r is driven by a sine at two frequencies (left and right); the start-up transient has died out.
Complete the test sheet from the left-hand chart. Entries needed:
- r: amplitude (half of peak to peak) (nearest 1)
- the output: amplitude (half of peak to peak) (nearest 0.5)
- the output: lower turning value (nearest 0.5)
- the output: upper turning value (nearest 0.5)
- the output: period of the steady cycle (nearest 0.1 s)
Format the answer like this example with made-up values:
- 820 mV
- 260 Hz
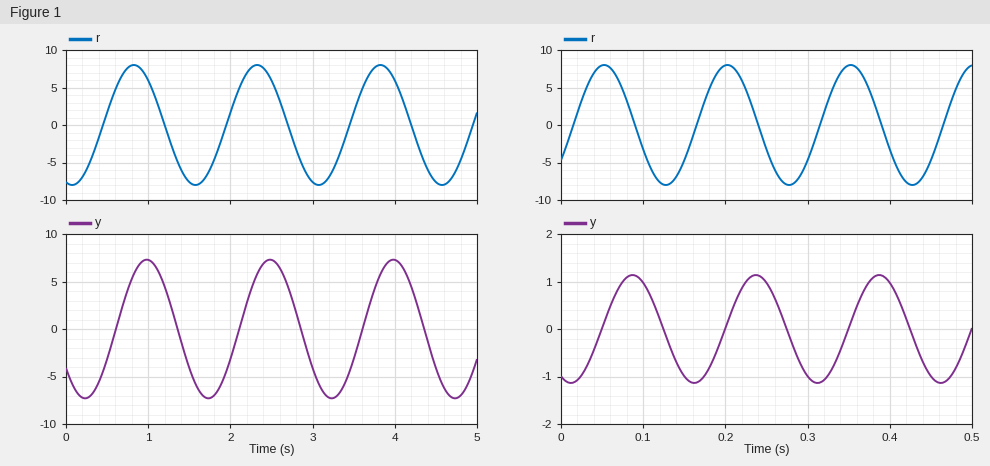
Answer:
- 8
- 7.5
- -7.5
- 7.5
- 1.5 s
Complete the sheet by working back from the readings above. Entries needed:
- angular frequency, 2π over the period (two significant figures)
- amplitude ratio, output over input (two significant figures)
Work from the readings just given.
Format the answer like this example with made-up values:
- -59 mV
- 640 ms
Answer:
- 4.2 rad/s
- 0.94
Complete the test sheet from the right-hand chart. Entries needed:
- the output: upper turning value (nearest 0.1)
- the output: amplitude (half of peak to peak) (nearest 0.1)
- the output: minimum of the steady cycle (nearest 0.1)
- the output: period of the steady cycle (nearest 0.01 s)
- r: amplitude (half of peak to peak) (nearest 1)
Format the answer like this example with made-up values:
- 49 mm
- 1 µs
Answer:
- 1.1
- 1.1
- -1.1
- 0.15 s
- 8
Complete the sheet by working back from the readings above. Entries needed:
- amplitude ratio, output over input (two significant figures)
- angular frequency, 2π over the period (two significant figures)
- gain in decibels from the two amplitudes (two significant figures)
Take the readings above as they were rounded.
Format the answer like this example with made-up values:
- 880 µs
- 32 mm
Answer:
- 0.14
- 42 rad/s
- -17 dB
